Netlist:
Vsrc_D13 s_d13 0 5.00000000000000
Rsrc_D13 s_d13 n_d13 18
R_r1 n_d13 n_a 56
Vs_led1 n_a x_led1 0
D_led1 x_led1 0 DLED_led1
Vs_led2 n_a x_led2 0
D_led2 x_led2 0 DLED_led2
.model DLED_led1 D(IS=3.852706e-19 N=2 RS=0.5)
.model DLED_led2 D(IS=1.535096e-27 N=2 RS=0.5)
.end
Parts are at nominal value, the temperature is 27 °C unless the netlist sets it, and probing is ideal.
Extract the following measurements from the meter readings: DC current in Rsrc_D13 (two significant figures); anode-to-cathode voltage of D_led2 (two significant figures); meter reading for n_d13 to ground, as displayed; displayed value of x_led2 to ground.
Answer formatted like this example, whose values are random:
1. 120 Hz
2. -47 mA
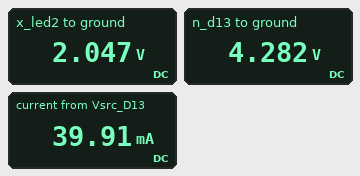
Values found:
1. 40 mA
2. 2.0 V
3. 4.282 V
4. 2.047 V
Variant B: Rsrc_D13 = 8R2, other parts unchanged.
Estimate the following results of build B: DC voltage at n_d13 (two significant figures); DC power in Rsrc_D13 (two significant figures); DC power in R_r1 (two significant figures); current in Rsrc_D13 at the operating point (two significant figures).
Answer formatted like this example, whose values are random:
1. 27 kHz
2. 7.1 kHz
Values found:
1. 4.6 V
2. 17 mW
3. 120 mW
4. 46 mA
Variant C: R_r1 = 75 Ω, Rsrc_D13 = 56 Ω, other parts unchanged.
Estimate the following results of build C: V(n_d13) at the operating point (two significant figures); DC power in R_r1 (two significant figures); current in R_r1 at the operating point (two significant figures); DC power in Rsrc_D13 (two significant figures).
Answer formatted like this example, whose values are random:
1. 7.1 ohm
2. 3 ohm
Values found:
1. 3.7 V
2. 39 mW
3. 23 mA
4. 29 mW
